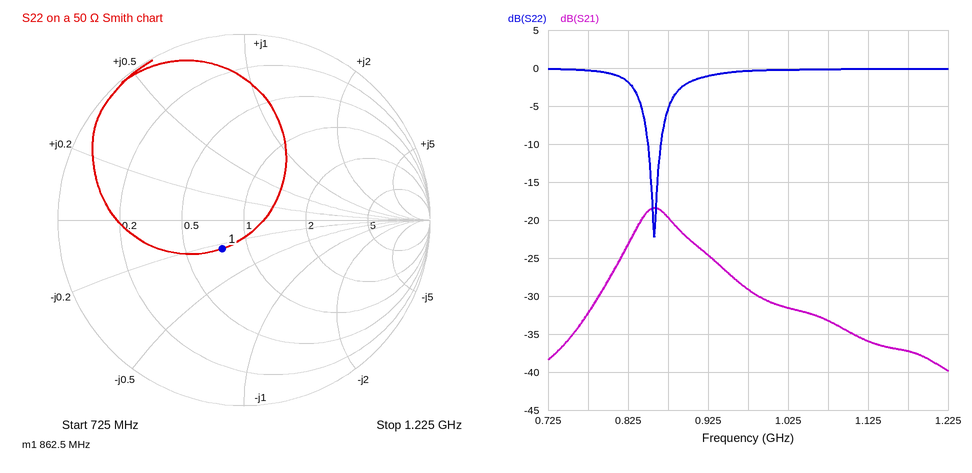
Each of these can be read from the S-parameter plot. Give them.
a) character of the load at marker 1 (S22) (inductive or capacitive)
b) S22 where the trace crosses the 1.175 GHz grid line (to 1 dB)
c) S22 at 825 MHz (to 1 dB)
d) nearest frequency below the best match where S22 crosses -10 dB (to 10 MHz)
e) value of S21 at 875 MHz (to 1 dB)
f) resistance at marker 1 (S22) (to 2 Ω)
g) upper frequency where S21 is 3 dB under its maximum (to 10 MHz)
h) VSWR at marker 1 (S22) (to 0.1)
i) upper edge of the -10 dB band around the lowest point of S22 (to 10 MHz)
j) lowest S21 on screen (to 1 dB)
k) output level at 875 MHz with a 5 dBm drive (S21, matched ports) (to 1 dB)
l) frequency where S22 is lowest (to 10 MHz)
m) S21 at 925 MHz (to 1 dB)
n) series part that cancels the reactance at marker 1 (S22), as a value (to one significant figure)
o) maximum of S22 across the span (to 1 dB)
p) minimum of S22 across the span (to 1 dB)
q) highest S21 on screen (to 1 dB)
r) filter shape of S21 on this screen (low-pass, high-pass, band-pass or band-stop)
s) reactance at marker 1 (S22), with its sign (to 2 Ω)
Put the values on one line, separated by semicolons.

capacitive; 0 dB; -2 dB; 850 MHz; -20 dB; 38 Ω; 890 MHz; 1.5; 870 MHz; -40 dB; -15 dBm; 860 MHz; -25 dB; 2 nH; 0 dB; -22 dB; -18 dB; band-pass; -12 Ω
